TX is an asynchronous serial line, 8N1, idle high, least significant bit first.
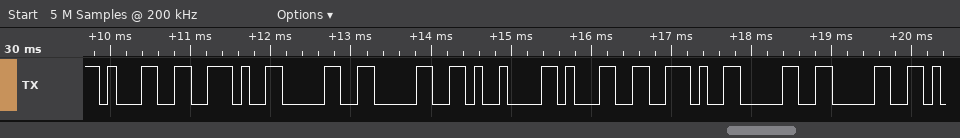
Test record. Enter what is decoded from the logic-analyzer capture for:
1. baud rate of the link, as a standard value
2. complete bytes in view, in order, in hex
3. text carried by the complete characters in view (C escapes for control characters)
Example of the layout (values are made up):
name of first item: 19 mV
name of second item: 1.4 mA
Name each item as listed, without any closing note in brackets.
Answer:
baud rate of the link, as a standard value: 9600 baud
complete bytes in view, in order, in hex: 0x31 0x2E 0x30 0x30 0x09 0x31 0x2E 0x30 0x30
text carried by the complete characters in view: "1.00\t1.00"
